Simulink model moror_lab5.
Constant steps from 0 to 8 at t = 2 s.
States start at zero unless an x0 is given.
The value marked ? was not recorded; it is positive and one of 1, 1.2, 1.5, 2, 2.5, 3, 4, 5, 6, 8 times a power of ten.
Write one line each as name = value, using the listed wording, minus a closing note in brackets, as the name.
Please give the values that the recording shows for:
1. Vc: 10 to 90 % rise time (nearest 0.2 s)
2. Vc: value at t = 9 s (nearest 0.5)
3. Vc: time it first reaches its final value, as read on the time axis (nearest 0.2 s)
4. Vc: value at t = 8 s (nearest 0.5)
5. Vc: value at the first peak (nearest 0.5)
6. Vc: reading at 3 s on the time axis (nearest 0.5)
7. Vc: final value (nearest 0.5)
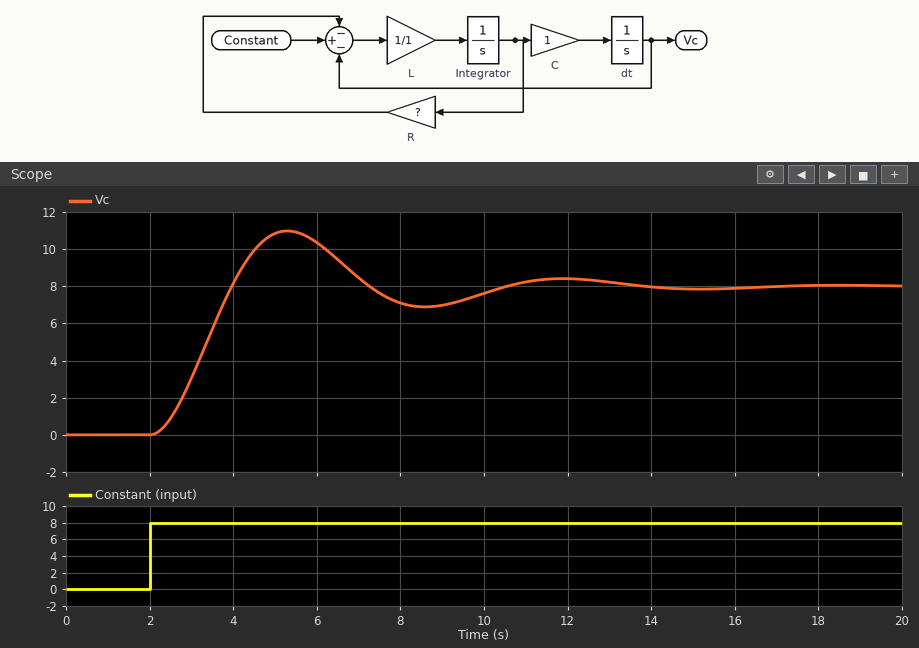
Vc: 10 to 90 % rise time = 1.4 s
Vc: value at t = 9 s = 7.0
Vc: time it first reaches its final value, as read on the time axis = 4.0 s
Vc: value at t = 8 s = 7.0
Vc: value at the first peak = 11.0
Vc: reading at 3 s on the time axis = 3.0
Vc: final value = 8.0
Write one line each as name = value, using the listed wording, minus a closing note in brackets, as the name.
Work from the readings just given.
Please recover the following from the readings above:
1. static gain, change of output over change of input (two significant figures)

static gain, change of output over change of input = 1.0
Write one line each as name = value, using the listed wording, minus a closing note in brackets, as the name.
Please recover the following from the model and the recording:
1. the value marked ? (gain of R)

the value marked ? = 0.6
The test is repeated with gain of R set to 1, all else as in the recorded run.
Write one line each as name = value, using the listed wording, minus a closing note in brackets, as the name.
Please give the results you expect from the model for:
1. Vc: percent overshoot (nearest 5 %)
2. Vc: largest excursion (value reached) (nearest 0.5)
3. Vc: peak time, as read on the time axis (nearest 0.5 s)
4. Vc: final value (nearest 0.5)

Vc: percent overshoot = 15 %
Vc: largest excursion (value reached) = 9.5
Vc: peak time, as read on the time axis = 5.5 s
Vc: final value = 8.0
